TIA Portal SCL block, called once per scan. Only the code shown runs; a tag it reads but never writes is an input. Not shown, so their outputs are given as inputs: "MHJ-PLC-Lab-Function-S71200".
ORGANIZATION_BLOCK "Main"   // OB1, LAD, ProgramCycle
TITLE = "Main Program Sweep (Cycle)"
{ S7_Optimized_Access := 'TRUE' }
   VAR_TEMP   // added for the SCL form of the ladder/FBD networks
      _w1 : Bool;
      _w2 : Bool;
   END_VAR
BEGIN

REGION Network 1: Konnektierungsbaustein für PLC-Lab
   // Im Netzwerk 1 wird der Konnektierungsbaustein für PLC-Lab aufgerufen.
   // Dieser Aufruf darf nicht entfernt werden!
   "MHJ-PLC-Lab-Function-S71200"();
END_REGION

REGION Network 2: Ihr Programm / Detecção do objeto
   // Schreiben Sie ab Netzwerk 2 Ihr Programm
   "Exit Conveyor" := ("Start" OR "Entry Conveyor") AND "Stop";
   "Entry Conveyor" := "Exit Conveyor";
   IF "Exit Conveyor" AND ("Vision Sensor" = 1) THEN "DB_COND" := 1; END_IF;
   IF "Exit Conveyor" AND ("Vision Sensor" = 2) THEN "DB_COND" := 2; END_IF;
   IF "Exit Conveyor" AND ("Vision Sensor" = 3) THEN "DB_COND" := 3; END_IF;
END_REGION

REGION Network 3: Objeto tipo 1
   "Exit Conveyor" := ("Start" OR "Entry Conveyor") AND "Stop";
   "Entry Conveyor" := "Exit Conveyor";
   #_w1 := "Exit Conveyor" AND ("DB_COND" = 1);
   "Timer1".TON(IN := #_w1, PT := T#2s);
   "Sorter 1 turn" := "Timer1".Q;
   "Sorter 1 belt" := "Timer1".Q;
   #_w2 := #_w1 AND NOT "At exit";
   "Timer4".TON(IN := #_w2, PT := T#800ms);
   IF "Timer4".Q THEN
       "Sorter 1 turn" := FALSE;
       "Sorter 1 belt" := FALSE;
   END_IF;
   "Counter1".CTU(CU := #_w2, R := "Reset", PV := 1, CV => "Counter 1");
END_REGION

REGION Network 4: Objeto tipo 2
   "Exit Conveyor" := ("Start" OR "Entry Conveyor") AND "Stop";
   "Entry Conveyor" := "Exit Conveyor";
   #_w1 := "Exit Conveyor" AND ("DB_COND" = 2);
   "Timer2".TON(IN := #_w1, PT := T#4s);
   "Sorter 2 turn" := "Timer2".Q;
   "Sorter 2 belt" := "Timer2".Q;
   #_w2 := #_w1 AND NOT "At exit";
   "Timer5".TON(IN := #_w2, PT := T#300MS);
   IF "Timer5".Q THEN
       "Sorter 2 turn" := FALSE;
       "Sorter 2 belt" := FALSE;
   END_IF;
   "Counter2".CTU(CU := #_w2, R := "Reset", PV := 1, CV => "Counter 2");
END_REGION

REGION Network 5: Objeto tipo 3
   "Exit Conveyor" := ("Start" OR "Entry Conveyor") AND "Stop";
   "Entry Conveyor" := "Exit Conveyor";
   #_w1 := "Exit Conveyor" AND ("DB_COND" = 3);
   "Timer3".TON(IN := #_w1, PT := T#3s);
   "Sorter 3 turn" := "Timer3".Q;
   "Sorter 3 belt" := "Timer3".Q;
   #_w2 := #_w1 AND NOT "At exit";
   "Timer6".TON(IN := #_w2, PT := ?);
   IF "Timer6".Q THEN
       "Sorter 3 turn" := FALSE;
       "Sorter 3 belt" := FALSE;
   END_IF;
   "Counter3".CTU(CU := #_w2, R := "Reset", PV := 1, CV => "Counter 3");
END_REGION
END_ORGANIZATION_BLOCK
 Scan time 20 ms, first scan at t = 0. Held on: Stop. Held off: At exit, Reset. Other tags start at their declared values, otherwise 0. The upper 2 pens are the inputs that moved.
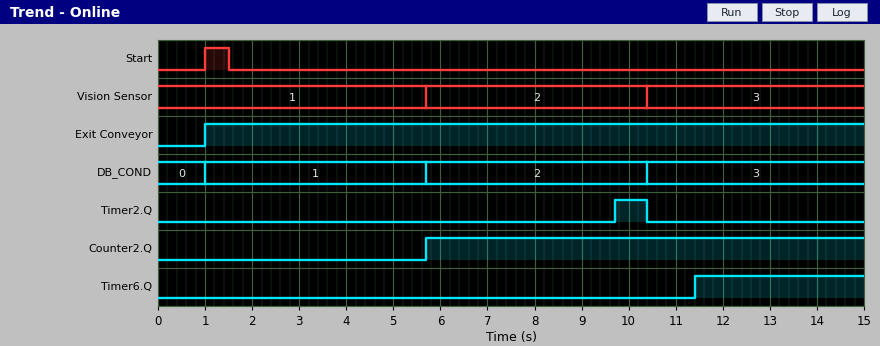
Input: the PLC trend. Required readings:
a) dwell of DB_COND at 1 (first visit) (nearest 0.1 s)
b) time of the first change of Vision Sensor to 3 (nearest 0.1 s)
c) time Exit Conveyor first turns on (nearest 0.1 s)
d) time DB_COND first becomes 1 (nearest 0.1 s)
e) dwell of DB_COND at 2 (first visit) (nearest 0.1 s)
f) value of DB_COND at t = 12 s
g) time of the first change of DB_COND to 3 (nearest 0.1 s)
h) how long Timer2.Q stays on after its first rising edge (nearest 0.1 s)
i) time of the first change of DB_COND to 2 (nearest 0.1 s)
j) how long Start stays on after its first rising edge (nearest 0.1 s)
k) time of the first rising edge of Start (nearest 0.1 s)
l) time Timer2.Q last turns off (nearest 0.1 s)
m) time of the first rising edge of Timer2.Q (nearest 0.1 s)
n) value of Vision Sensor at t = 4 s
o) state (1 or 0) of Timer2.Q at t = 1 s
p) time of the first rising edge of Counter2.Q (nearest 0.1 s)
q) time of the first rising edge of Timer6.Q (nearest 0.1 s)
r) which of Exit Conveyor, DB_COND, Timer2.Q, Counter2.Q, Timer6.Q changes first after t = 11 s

4.7 s
10.4 s
1.0 s
1.0 s
4.7 s
3
10.4 s
0.7 s
5.7 s
0.5 s
1.0 s
10.4 s
9.7 s
1
0
5.7 s
11.4 s
Timer6.Q
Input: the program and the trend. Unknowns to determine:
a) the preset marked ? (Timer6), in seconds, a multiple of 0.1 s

1.0 s
